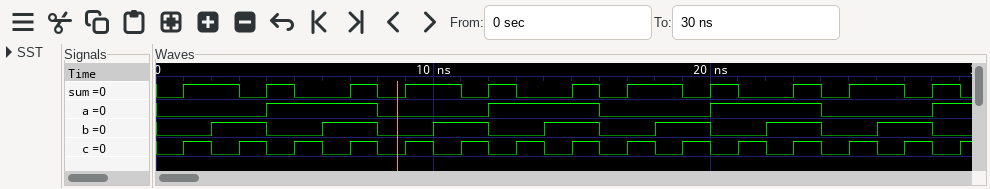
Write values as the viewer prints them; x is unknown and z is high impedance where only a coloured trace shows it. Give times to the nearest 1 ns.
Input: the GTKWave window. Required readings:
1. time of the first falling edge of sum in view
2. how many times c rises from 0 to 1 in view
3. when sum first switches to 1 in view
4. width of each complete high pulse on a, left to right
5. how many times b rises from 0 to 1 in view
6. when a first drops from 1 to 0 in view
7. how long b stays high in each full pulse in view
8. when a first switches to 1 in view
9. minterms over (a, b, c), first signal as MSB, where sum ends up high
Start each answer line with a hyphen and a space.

- 3 ns
- 15
- 1 ns
- 4 ns, 4 ns, 4 ns
- 7
- 8 ns
- 2 ns, 2 ns, 2 ns, 2 ns, 2 ns, 2 ns, 2 ns
- 4 ns
- 1, 2, 4, 7
